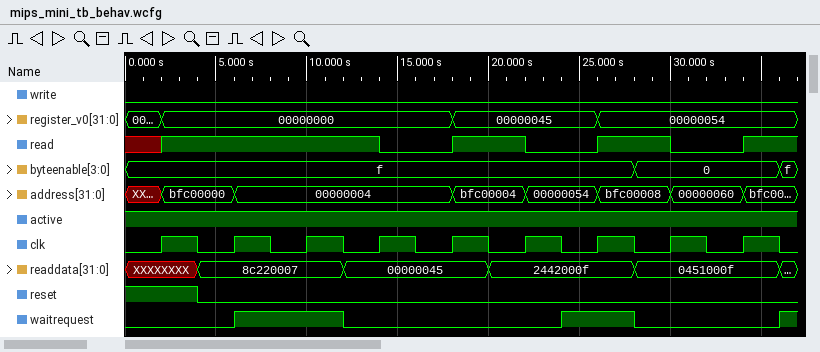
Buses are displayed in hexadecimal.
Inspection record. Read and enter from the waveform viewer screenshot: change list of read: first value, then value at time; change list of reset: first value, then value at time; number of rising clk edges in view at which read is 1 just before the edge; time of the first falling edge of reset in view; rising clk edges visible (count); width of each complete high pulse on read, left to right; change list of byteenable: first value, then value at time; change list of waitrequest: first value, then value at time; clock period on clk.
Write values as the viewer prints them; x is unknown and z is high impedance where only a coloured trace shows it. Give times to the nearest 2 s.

x, 1 at 2 s, 0 at 14 s, 1 at 18 s, 0 at 22 s, 1 at 26 s, 0 at 30 s, 1 at 34 s
1, 0 at 4 s
5
4 s
9
4 s, 4 s
f, 0 at 28 s, f at 36 s
0, 1 at 6 s, 0 at 12 s, 1 at 24 s, 0 at 28 s, 1 at 36 s
4 s
